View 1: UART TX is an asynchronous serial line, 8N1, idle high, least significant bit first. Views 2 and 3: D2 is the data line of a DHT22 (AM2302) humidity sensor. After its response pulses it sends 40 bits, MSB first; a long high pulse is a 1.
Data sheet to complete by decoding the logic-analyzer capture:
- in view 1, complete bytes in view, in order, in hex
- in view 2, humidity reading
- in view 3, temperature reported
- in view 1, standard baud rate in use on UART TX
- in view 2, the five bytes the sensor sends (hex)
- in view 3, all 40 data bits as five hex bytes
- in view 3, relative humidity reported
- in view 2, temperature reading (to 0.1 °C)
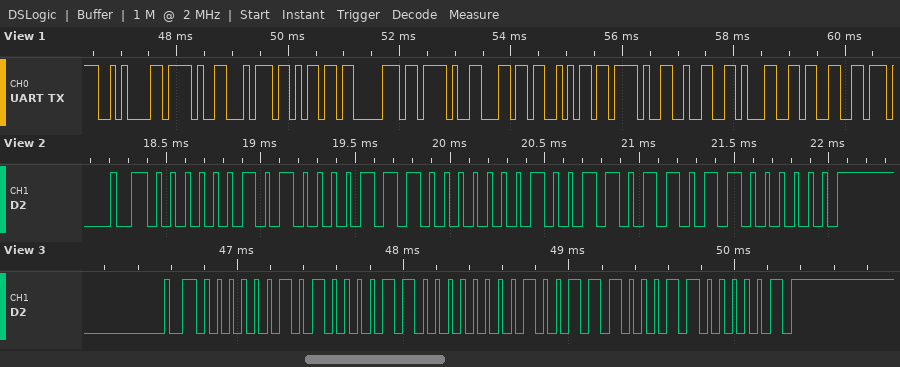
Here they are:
0A 2F 74 6D 70 2F 6C 6A 2F 32 31 33
64.7 %
31.2 °C
9600 baud
02 87 01 36 C0
02 86 01 38 C1
64.6 %
31.0 °C
